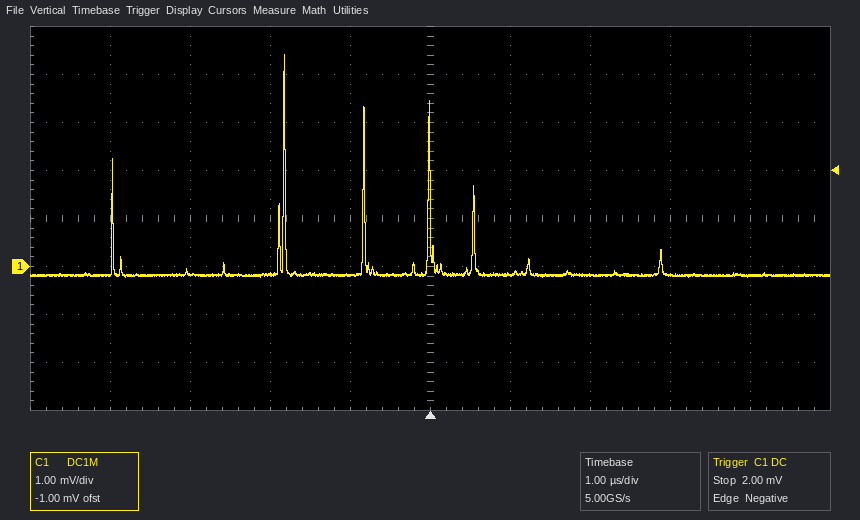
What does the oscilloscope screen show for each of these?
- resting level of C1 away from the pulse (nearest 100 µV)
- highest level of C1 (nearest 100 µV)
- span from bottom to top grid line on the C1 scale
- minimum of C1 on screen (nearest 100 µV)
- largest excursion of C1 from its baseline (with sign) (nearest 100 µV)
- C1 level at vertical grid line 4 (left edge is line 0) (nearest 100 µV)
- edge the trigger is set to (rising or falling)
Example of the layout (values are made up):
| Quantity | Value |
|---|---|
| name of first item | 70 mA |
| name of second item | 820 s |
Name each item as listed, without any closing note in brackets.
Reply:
| Quantity | Value |
|---|---|
| resting level of C1 away from the pulse | -200 µV |
| highest level of C1 | 4.4 mV |
| span from bottom to top grid line on the C1 scale | 8 mV |
| minimum of C1 on screen | -200 µV |
| largest excursion of C1 from its baseline (with sign) | +4.6 mV |
| C1 level at vertical grid line 4 (left edge is line 0) | -200 µV |
| edge the trigger is set to | falling |
